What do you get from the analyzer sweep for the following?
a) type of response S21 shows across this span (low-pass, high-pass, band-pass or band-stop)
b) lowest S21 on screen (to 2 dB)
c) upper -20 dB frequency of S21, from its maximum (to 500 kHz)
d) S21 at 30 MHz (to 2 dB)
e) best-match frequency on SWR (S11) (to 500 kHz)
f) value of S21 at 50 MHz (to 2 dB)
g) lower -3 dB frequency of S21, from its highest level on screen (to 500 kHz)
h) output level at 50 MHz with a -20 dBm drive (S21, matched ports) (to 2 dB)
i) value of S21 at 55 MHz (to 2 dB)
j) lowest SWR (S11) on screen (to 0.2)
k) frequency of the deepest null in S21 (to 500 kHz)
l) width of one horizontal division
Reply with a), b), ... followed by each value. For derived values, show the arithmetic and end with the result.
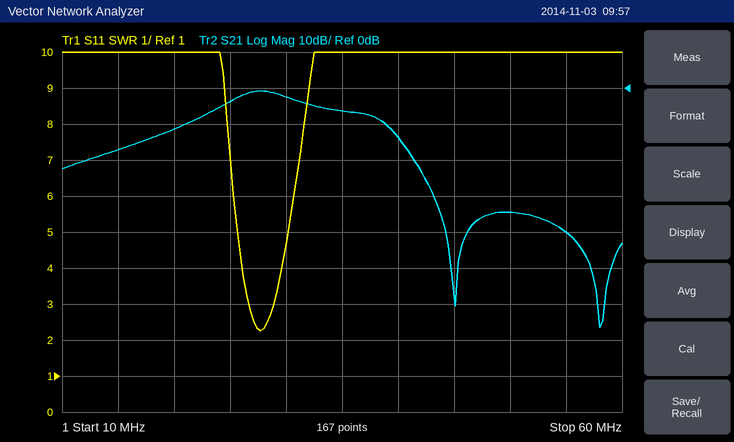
a) band-pass
b) -66 dB
c) 41.5 MHz
d) -2 dB
e) 27.5 MHz
f) -34 dB
g) 25.0 MHz
h) -20 dBm + (-34 dB) = -54 dBm
i) -40 dB
j) 2.2
k) 58.0 MHz
l) 5 MHz
